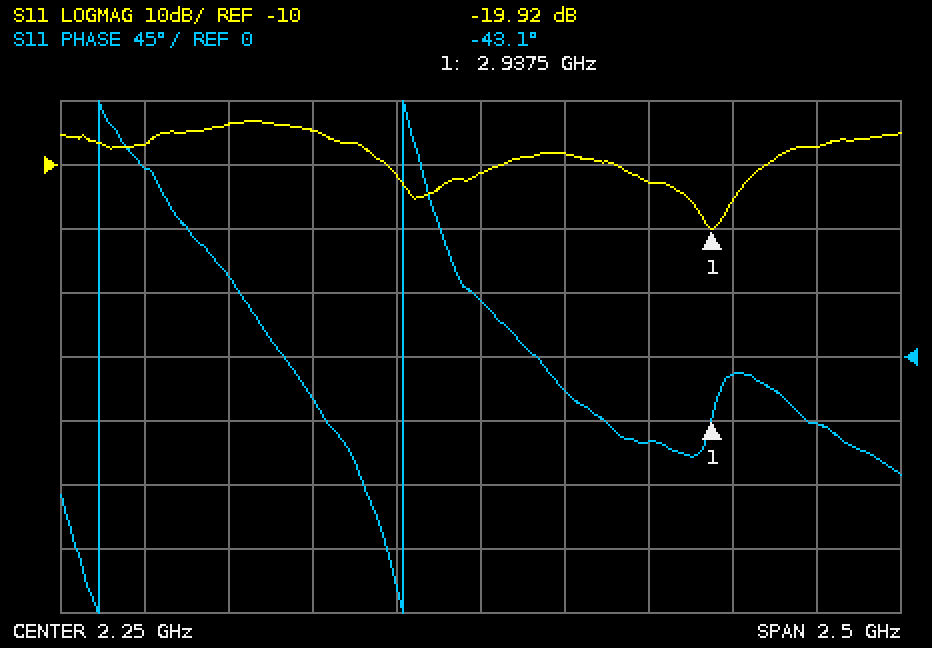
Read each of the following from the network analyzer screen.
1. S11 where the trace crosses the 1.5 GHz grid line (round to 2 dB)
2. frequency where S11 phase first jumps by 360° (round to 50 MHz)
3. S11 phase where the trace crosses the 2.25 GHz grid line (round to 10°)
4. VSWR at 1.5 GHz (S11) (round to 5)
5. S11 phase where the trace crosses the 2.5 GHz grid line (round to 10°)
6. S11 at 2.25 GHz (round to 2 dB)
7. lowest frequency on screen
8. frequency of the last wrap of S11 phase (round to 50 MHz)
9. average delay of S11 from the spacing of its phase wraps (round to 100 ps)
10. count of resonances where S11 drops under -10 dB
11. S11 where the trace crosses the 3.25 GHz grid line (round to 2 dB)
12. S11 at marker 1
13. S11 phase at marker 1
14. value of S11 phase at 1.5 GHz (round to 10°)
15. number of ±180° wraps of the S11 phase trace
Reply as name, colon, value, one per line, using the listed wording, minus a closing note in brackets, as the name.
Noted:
S11 where the trace crosses the 1.5 GHz grid line: -4 dB
frequency where S11 phase first jumps by 360°: 1.10 GHz
S11 phase where the trace crosses the 2.25 GHz grid line: 40°
VSWR at 1.5 GHz (S11): 5
S11 phase where the trace crosses the 2.5 GHz grid line: -20°
S11 at 2.25 GHz: -12 dB
lowest frequency on screen: 1 GHz
frequency of the last wrap of S11 phase: 2.00 GHz
average delay of S11 from the spacing of its phase wraps: 1.1 ns
count of resonances where S11 drops under -10 dB: 2
S11 where the trace crosses the 3.25 GHz grid line: -8 dB
S11 at marker 1: -19.92 dB
S11 phase at marker 1: -43.1°
value of S11 phase at 1.5 GHz: 60°
number of ±180° wraps of the S11 phase trace: 2
